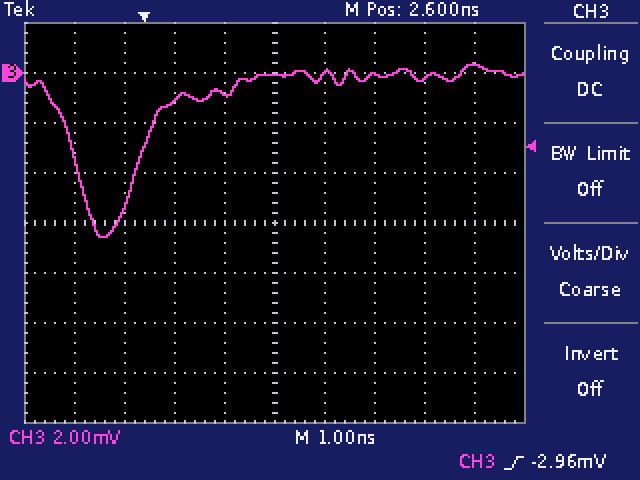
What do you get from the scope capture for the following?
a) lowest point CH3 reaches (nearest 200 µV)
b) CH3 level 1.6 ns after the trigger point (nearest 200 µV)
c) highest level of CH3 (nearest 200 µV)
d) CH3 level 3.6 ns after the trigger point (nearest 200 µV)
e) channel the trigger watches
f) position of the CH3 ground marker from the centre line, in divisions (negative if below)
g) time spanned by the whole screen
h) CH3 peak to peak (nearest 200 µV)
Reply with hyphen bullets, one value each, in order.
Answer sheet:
- -6.6 mV
- -800 µV
- 400 µV
- 0.0 mV
- CH3
- +3.0 div
- 10 ns
- 7.0 mV
